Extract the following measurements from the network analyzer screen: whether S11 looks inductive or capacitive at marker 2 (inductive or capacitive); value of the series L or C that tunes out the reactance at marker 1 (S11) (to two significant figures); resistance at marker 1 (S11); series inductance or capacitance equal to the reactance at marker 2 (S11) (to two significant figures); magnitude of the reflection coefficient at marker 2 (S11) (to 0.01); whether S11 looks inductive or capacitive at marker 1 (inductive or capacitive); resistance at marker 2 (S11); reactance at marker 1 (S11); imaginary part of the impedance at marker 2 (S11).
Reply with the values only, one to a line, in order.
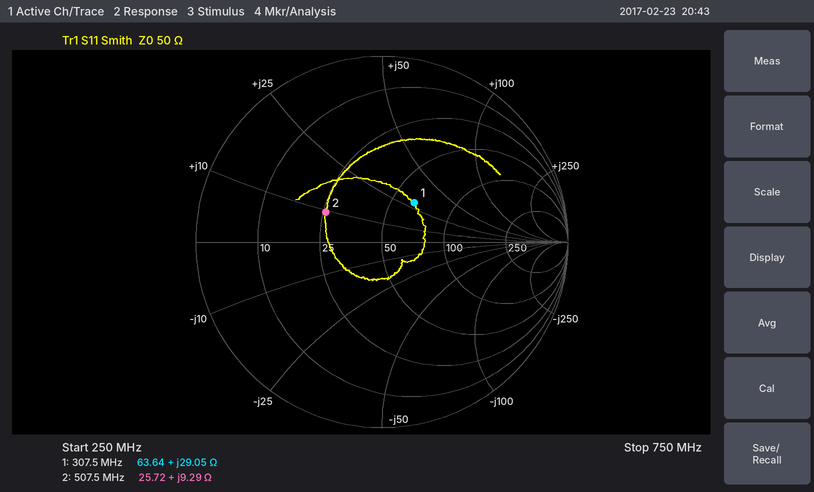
inductive
18 pF
63.64 Ω
2.9 nH
0.34
inductive
25.72 Ω
+29.05 Ω
+9.29 Ω
